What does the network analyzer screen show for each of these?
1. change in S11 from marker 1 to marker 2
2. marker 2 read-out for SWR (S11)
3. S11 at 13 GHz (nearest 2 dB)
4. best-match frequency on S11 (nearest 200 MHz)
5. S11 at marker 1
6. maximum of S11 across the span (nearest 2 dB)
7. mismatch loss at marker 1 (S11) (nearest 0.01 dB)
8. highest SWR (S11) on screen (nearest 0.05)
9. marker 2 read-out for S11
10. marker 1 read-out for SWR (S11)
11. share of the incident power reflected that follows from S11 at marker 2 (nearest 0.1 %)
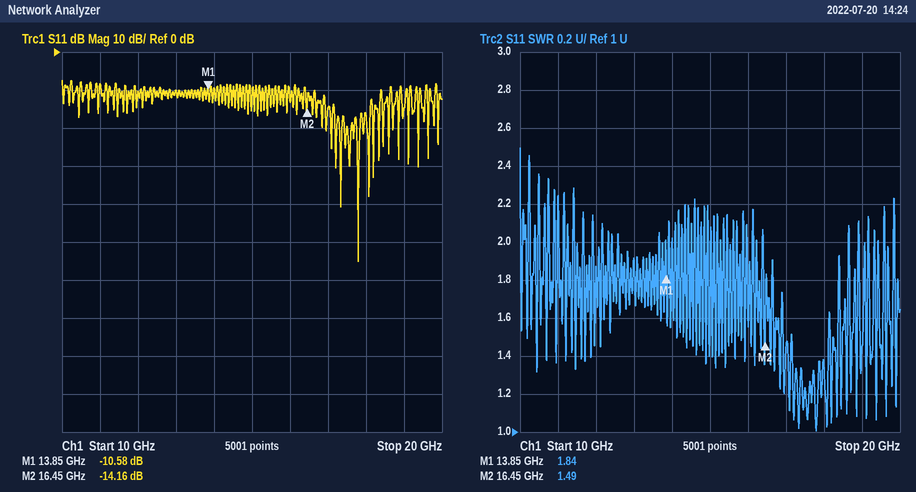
-3.58 dB
1.49
-10 dB
17.8 GHz
-10.58 dB
-8 dB
0.40 dB
2.50
-14.16 dB
1.84
3.8 %
